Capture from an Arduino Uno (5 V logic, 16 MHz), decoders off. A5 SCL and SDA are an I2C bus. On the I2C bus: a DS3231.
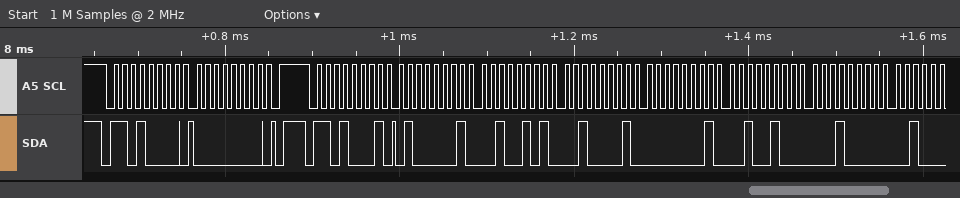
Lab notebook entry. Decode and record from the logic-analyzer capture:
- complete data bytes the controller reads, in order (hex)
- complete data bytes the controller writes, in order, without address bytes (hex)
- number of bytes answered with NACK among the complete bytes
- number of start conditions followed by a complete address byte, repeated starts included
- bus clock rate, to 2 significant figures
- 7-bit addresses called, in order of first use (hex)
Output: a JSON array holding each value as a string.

["41 25 21 01 24 10", "00", "0", "2", "100 kHz", "0x68"]
